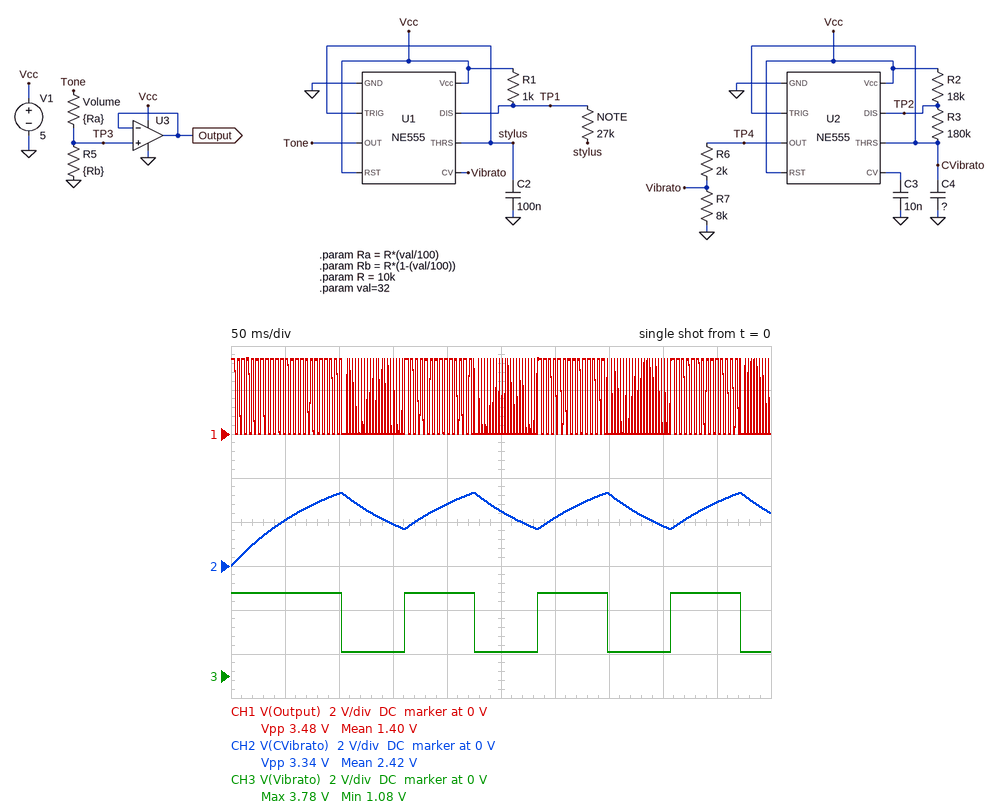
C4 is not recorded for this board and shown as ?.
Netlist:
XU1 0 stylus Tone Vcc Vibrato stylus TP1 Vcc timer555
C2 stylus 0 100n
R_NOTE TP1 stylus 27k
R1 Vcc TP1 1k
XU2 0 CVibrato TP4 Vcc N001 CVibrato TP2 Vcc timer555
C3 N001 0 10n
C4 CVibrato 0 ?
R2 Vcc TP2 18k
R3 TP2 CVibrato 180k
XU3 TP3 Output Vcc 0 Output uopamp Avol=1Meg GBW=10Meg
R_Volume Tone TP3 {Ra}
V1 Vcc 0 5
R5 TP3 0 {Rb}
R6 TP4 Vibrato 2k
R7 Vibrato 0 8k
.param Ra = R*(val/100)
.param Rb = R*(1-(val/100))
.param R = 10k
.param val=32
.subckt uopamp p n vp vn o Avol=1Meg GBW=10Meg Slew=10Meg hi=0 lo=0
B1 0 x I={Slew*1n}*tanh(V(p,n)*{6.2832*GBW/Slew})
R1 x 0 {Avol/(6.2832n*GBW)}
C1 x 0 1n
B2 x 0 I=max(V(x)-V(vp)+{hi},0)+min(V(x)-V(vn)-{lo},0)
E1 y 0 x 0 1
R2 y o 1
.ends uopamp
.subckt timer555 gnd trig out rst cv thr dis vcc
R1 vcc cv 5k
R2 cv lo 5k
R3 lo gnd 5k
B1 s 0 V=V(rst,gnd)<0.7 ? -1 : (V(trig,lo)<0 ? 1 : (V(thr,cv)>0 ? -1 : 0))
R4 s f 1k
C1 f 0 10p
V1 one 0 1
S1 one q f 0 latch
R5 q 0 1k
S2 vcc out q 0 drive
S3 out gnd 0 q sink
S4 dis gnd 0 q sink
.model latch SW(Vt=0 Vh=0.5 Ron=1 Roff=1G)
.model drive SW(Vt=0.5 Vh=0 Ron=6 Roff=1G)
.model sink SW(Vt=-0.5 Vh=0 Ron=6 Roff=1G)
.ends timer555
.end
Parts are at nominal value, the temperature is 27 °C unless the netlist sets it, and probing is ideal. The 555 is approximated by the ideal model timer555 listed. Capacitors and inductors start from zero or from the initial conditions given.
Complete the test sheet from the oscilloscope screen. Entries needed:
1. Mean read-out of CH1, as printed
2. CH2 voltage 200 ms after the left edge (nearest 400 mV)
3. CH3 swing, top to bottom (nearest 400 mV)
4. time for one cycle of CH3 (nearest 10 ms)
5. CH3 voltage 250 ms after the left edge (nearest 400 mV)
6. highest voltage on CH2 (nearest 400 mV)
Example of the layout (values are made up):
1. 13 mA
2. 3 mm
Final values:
1. 1.40 V
2. 2.8 V
3. 2.8 V
4. 120 ms
5. 1.2 V
6. 3.2 V
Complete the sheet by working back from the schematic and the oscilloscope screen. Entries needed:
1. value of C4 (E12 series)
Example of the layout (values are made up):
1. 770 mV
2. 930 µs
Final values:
1. 470 nF
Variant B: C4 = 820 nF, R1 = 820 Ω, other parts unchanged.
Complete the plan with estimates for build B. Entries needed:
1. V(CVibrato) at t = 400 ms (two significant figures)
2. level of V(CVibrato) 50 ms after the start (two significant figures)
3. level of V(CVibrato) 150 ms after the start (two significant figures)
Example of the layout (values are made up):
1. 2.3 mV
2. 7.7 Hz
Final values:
1. 3.2 V
2. 1.3 V
3. 3.0 V
